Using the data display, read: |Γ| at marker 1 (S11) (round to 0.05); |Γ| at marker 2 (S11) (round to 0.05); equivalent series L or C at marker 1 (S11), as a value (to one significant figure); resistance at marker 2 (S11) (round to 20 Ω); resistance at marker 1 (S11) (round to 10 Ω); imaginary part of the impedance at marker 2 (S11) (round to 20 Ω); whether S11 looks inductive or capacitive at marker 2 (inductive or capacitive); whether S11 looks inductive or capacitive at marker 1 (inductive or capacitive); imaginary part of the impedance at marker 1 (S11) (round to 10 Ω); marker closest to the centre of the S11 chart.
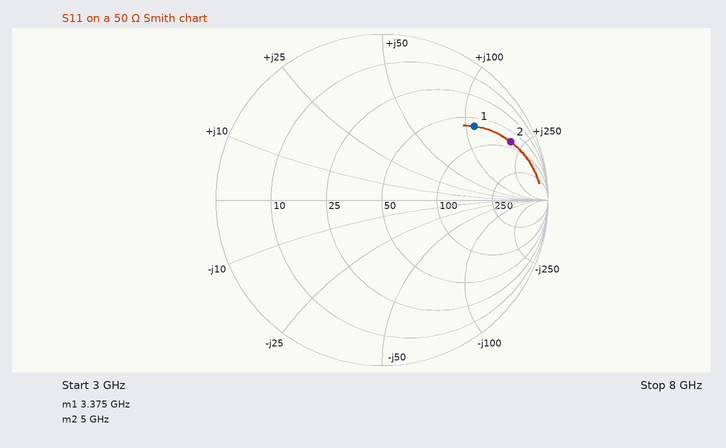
0.70
0.85
5 nH
80 Ω
60 Ω
+200 Ω
inductive
inductive
+110 Ω
marker 1
